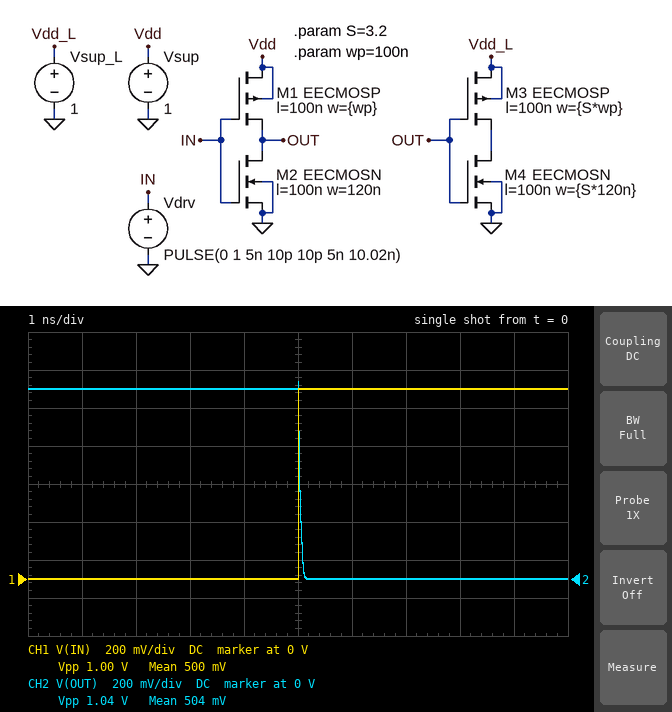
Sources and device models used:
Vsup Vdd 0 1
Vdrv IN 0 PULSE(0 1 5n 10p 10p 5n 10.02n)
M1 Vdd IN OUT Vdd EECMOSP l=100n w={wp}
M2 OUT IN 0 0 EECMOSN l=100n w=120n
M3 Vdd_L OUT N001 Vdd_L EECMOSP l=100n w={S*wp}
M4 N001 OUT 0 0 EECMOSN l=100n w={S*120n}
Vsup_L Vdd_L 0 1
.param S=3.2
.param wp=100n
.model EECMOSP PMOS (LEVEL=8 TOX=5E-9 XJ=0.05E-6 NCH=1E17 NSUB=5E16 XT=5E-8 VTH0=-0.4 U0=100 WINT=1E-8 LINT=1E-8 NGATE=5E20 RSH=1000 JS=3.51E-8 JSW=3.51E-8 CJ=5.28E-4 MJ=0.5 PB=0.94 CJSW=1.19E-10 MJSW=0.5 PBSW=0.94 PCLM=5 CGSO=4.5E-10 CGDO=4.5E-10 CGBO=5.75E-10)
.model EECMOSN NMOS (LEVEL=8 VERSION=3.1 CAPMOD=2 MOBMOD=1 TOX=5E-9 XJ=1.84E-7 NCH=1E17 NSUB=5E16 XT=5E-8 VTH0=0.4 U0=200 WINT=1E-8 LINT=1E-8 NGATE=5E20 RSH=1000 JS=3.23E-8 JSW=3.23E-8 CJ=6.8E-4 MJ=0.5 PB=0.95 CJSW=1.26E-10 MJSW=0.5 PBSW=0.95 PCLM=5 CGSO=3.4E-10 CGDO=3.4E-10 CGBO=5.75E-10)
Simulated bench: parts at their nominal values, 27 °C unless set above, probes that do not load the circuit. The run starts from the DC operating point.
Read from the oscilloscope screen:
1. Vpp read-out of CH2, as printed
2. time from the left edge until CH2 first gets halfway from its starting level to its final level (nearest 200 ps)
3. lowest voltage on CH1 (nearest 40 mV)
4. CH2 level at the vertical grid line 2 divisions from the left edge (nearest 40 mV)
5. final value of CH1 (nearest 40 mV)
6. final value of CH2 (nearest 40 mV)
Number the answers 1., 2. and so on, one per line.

1. 1.04 V
2. 5.0 ns
3. 0 V
4. 1.00 V
5. 1.00 V
6. 0 V
